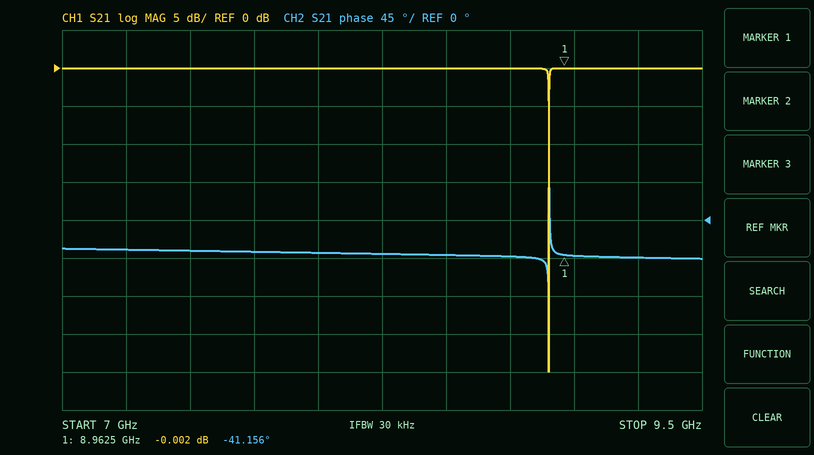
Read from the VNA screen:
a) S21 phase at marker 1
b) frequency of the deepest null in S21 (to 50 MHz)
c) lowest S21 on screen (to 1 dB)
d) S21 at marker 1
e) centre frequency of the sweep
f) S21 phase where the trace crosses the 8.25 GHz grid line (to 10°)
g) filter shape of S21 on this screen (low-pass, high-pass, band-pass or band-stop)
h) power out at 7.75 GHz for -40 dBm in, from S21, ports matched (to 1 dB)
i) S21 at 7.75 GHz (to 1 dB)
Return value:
-41.156°
8.90 GHz
-40 dB
-0.002 dB
8.25 GHz
-40°
band-stop
-40 dBm
0 dB
